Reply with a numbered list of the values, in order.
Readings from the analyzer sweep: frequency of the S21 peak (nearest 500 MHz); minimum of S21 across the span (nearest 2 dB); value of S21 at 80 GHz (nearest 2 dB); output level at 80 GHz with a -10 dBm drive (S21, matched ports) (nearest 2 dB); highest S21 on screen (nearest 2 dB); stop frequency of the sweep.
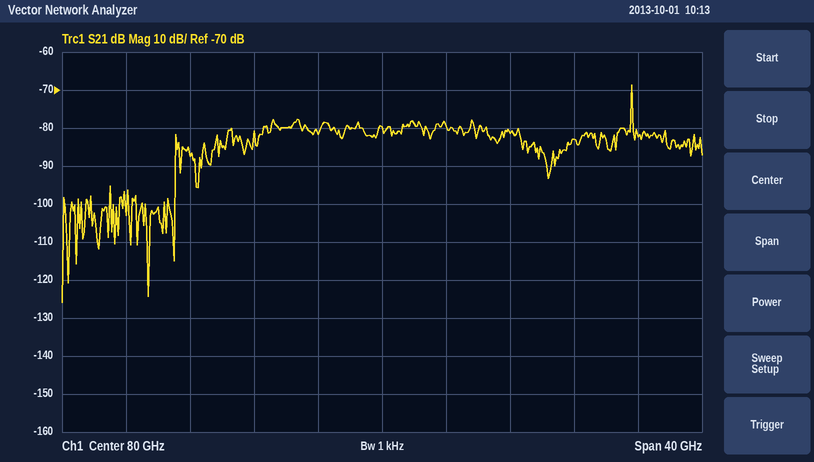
1. 95.5 GHz
2. -126 dB
3. -80 dB
4. -90 dBm
5. -68 dB
6. 100 GHz
